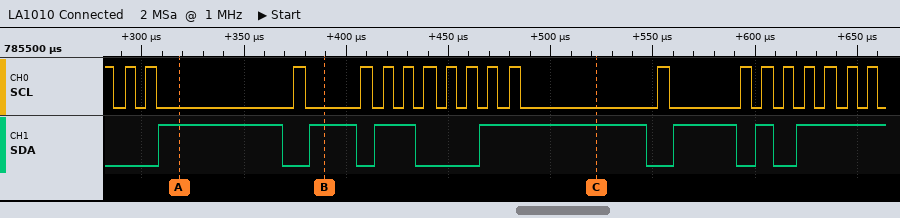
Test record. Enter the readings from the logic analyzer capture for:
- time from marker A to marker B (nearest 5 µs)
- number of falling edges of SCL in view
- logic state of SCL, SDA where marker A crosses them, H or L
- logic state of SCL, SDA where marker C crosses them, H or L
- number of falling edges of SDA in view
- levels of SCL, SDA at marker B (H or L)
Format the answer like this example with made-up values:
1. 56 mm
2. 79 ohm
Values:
1. 70 µs
2. 20
3. SCL=L, SDA=H
4. SCL=L, SDA=H
5. 6
6. SCL=L, SDA=H
